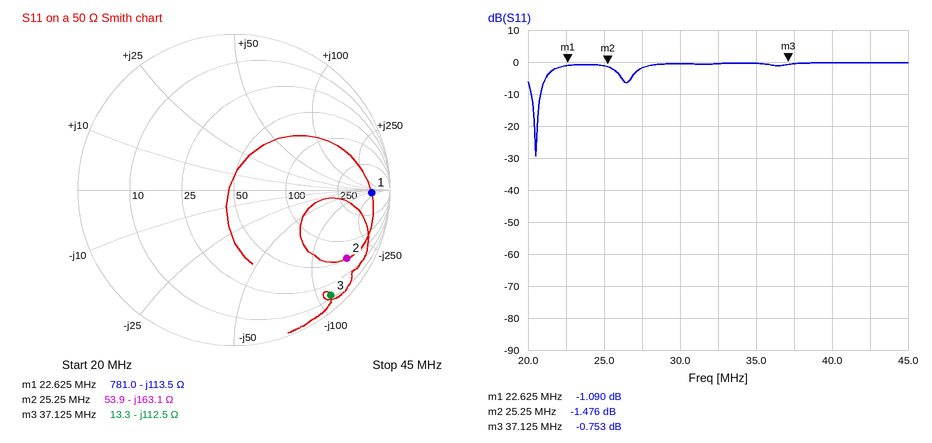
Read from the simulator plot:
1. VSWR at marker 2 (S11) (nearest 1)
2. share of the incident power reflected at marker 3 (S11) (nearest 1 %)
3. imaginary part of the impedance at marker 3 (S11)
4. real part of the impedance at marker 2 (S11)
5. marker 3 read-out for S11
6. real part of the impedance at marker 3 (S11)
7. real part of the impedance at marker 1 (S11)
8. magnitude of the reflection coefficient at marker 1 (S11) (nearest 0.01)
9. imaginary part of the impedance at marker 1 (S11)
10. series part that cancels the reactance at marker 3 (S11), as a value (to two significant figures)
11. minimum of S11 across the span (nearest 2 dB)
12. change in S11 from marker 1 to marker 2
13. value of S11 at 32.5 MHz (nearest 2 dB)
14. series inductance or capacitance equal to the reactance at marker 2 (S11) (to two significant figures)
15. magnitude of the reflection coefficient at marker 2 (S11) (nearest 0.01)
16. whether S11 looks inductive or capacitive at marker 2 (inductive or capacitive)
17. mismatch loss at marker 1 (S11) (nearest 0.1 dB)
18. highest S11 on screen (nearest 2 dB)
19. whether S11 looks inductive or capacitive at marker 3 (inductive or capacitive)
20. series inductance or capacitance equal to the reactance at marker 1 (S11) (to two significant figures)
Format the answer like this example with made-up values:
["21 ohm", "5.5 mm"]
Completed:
["12", "84 %", "-112.5 Ω", "53.9 Ω", "-0.753 dB", "13.3 Ω", "781.0 Ω", "0.88", "-113.5 Ω", "480 nH", "-30 dB", "-0.386 dB", "0 dB", "39 pF", "0.84", "capacitive", "6.5 dB", "0 dB", "capacitive", "62 pF"]
